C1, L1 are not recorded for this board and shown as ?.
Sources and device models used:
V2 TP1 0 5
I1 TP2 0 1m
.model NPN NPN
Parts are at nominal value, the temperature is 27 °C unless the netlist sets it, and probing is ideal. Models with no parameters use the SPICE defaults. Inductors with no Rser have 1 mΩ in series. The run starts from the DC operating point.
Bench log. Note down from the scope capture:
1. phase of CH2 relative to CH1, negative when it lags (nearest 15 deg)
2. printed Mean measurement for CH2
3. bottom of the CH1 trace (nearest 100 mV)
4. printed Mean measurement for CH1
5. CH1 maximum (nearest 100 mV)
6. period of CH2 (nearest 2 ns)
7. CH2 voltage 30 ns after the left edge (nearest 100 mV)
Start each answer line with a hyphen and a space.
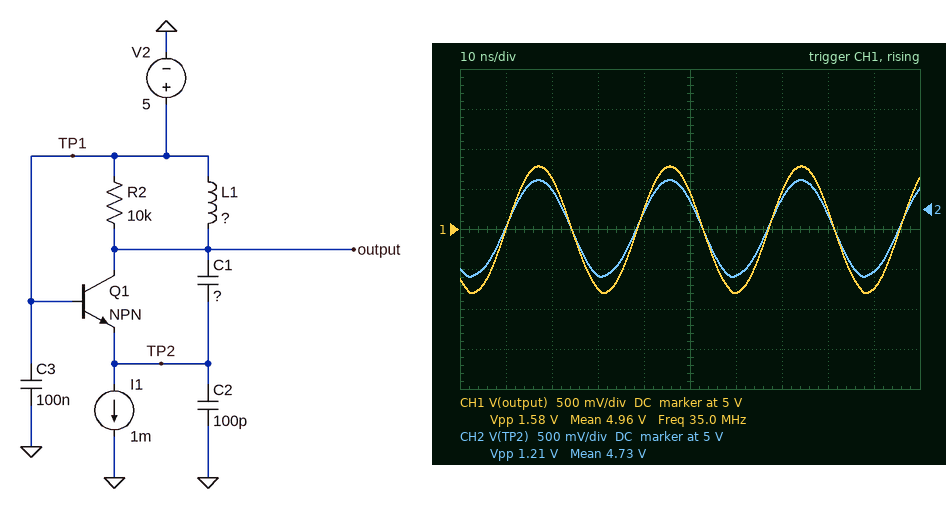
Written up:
- 0 deg
- 4.73 V
- 4.2 V
- 4.96 V
- 5.8 V
- 28 ns
- 4.2 V
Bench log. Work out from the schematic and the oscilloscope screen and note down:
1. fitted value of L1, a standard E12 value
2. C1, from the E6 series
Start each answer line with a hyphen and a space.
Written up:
- 270 nH
- 330 pF
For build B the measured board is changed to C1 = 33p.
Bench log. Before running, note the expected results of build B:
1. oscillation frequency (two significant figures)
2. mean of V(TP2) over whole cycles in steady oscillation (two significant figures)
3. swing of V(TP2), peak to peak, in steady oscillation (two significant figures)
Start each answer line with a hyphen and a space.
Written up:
- 62 MHz
- 4.4 V
- 400 mV
